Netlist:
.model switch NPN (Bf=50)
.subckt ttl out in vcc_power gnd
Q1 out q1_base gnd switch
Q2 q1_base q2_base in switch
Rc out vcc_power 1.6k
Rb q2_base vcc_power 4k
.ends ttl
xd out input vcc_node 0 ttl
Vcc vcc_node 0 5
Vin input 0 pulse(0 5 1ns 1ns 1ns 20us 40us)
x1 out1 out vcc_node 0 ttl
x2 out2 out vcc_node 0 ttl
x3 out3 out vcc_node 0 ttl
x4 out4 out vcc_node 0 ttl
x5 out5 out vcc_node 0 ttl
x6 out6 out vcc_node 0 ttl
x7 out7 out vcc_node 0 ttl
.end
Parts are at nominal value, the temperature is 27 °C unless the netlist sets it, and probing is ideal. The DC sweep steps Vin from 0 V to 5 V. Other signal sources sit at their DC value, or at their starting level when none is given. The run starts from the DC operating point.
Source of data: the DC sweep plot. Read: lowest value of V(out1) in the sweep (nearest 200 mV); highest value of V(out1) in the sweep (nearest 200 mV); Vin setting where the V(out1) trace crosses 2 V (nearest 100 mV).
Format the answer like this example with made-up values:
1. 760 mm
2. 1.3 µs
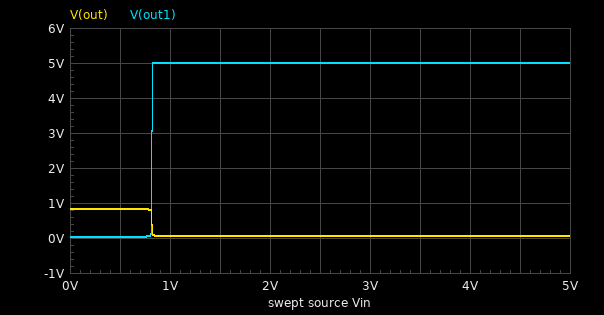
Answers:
1. 0 V
2. 5.0 V
3. 800 mV
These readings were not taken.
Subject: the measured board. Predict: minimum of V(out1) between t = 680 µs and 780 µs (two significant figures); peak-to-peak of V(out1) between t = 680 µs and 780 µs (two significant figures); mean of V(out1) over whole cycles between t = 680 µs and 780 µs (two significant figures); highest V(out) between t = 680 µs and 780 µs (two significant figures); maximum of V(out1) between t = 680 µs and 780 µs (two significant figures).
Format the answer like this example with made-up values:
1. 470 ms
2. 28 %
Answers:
1. 40 mV
2. 5.0 V
3. 2.5 V
4. 830 mV
5. 5.0 V
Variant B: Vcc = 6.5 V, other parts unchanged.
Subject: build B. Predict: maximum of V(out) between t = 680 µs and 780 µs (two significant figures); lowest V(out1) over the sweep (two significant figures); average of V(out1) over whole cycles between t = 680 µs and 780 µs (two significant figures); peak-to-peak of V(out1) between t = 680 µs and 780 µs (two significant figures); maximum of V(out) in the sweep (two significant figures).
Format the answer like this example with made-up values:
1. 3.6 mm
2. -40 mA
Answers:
1. 840 mV
2. 39 mV
3. 3.3 V
4. 6.5 V
5. 840 mV
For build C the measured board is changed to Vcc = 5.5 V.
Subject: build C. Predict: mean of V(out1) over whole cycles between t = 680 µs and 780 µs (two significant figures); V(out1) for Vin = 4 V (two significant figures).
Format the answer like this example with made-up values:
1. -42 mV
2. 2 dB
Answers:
1. 2.8 V
2. 5.5 V
